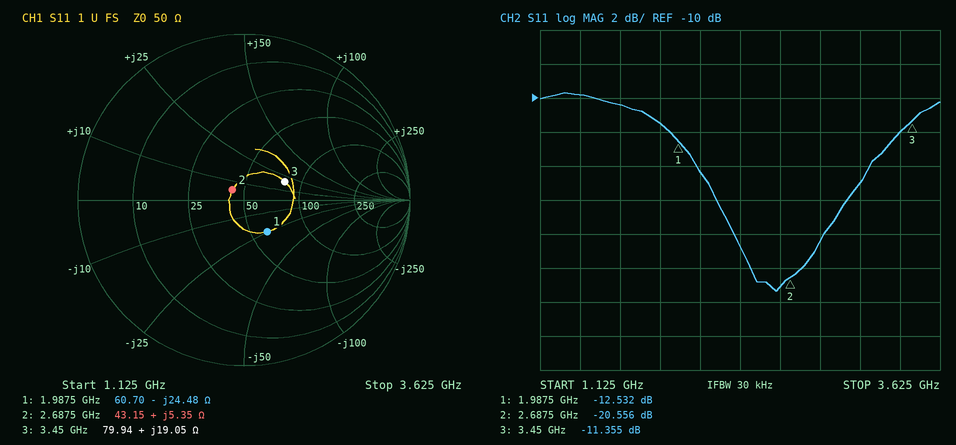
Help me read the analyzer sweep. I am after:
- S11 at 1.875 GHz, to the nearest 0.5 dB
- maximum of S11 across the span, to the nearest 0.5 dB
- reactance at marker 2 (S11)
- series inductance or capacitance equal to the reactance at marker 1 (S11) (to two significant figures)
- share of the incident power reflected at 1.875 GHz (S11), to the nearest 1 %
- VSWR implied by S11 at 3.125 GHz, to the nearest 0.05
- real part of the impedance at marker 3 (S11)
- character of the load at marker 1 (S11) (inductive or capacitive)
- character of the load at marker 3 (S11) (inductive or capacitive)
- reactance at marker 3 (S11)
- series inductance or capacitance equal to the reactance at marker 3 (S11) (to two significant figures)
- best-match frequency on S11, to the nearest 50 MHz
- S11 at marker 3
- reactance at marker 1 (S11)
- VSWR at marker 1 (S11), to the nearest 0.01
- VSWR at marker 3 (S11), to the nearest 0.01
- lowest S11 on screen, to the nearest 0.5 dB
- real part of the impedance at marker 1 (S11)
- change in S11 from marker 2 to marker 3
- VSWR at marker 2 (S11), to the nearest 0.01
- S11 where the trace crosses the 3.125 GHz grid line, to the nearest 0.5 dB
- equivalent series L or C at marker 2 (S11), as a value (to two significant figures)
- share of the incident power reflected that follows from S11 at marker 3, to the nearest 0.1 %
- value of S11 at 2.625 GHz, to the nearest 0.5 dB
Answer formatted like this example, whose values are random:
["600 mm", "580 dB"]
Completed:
["-11.5 dB", "-9.5 dB", "+5.35 Ω", "3.3 pF", "7 %", "1.45", "79.94 Ω", "capacitive", "inductive", "+19.05 Ω", "880 pH", "2.60 GHz", "-11.355 dB", "-24.48 Ω", "1.62", "1.74", "-21.5 dB", "60.70 Ω", "9.201 dB", "1.21", "-15.0 dB", "320 pH", "7.3 %", "-21.0 dB"]
